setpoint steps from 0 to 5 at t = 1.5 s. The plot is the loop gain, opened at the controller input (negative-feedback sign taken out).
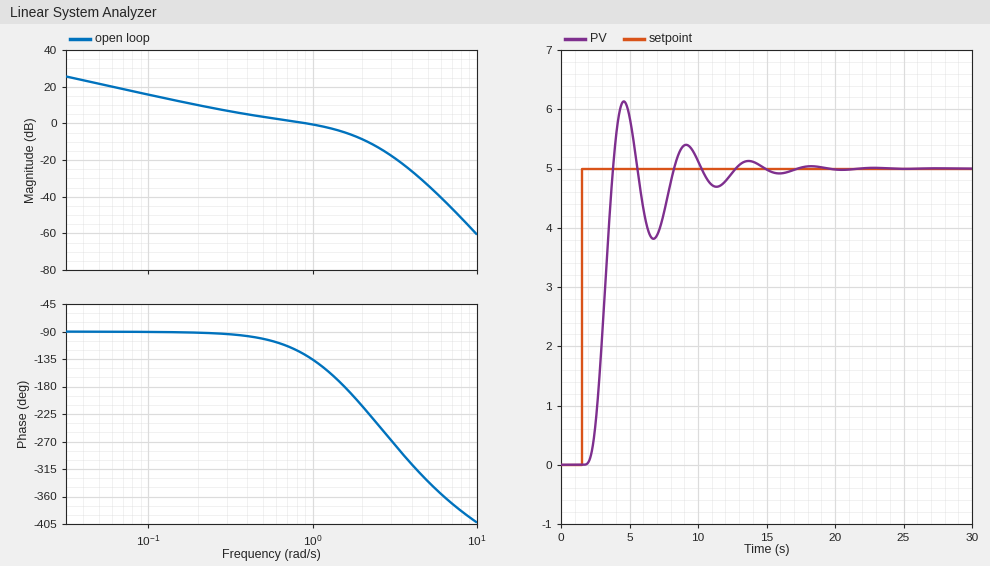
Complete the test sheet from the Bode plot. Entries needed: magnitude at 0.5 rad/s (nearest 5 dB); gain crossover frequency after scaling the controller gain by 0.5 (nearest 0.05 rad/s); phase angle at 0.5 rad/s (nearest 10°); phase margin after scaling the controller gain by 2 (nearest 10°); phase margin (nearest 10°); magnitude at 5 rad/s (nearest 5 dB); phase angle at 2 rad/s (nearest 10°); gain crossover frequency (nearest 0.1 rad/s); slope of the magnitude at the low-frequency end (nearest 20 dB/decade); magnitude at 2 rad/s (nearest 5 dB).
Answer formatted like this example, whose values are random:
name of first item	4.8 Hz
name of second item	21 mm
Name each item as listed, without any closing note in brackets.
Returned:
magnitude at 0.5 rad/s	5 dB
gain crossover frequency after scaling the controller gain by 0.5	0.35 rad/s
phase angle at 0.5 rad/s	-100°
phase margin after scaling the controller gain by 2	-10°
phase margin	50°
magnitude at 5 rad/s	-35 dB
phase angle at 2 rad/s	-210°
gain crossover frequency	0.9 rad/s
slope of the magnitude at the low-frequency end	-20 dB/decade
magnitude at 2 rad/s	-10 dB
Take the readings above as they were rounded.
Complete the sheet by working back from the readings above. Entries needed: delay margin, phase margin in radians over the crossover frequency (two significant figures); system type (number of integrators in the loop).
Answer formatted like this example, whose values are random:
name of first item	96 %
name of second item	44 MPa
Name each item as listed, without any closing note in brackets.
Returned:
delay margin, phase margin in radians over the crossover frequency	0.97 s
system type	1
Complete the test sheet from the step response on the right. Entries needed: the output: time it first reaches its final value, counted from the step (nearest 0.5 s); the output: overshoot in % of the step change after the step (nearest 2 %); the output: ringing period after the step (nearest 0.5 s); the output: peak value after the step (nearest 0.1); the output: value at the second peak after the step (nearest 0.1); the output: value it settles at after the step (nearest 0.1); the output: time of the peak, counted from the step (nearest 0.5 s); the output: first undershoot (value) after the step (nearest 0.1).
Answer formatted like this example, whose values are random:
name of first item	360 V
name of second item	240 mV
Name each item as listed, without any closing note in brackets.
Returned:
the output: time it first reaches its final value, counted from the step	2.5 s
the output: overshoot in % of the step change after the step	22 %
the output: ringing period after the step	4.5 s
the output: peak value after the step	6.1
the output: value at the second peak after the step	5.4
the output: value it settles at after the step	5.0
the output: time of the peak, counted from the step	3.0 s
the output: first undershoot (value) after the step	3.8
